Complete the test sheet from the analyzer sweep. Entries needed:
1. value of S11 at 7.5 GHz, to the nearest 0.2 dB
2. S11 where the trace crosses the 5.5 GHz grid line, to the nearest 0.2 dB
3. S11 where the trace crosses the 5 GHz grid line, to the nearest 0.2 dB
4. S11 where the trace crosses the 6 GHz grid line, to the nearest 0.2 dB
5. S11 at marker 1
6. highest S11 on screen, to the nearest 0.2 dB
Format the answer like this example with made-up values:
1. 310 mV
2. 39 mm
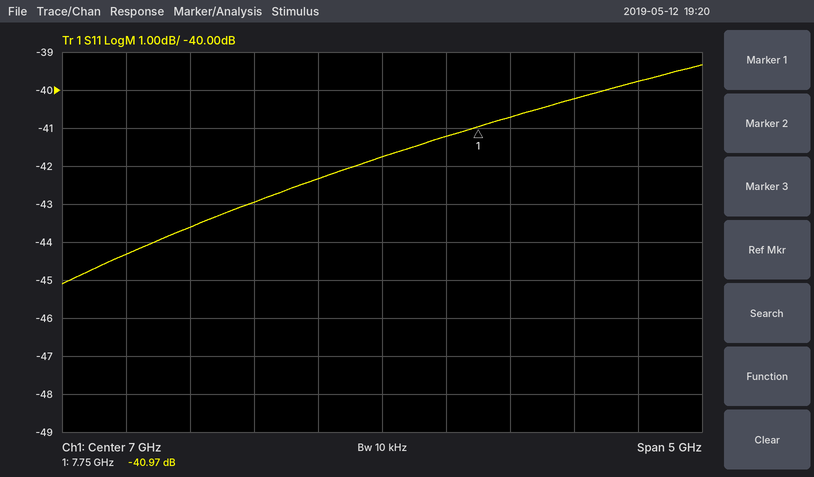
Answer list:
1. -41.2 dB
2. -43.6 dB
3. -44.4 dB
4. -43.0 dB
5. -40.97 dB
6. -39.4 dB
